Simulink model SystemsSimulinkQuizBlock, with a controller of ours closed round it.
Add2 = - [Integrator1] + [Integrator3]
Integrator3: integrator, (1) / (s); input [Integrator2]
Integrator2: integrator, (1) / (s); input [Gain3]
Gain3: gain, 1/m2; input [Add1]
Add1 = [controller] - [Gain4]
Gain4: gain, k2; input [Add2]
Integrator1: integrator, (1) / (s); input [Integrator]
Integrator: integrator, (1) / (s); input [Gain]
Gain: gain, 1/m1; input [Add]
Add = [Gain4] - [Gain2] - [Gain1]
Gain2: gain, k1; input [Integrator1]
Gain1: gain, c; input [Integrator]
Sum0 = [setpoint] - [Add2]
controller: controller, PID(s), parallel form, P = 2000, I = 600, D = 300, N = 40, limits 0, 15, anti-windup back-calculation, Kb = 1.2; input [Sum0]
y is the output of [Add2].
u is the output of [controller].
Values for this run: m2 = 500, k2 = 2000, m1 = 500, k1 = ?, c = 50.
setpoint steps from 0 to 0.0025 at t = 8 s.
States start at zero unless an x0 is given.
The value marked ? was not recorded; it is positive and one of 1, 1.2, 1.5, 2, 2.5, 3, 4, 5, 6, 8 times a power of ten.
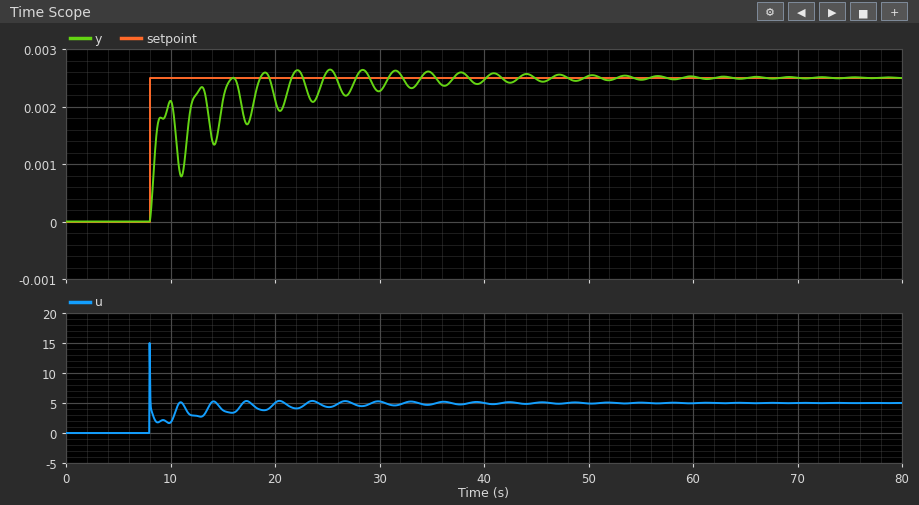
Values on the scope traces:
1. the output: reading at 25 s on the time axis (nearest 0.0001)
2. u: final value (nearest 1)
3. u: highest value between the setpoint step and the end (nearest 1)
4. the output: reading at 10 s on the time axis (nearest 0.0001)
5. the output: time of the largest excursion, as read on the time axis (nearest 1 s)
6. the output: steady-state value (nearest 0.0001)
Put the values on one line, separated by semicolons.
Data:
0.0026; 5; 15; 0.0021; 25 s; 0.0025
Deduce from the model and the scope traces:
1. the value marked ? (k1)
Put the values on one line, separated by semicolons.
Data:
4000
